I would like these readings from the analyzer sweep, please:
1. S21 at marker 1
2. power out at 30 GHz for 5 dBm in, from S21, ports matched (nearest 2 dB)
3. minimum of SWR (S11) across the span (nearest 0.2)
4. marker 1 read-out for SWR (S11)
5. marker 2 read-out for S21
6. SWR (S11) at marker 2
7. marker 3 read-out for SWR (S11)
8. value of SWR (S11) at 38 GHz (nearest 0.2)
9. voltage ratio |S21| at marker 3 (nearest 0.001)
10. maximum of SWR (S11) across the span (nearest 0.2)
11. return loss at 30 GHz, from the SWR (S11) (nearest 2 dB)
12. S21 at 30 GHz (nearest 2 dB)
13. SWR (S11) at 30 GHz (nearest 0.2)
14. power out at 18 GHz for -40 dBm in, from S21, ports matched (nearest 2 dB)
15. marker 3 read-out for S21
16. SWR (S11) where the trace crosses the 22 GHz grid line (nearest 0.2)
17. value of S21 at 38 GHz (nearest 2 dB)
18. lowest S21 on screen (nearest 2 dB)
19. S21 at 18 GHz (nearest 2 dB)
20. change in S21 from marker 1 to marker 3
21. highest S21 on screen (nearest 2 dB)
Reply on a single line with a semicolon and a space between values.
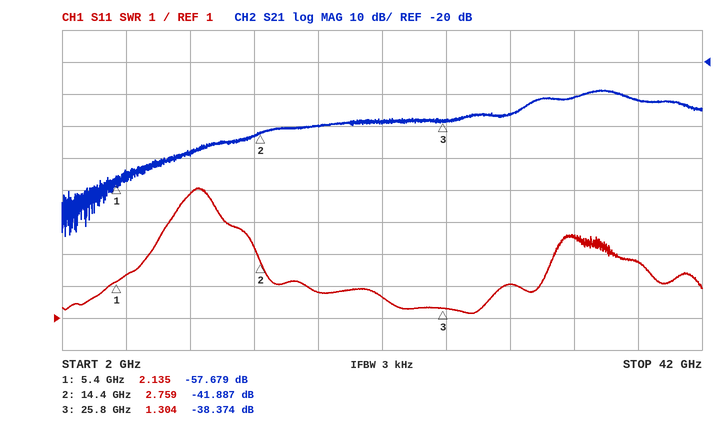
-57.679 dB; -32 dBm; 1.2; 2.135; -41.887 dB; 2.759; 1.304; 2.8; 0.012; 5.0; 10 dB; -36 dB; 2.0; -80 dBm; -38.374 dB; 1.6; -32 dB; -74 dB; -40 dB; 19.305 dB; -28 dB
